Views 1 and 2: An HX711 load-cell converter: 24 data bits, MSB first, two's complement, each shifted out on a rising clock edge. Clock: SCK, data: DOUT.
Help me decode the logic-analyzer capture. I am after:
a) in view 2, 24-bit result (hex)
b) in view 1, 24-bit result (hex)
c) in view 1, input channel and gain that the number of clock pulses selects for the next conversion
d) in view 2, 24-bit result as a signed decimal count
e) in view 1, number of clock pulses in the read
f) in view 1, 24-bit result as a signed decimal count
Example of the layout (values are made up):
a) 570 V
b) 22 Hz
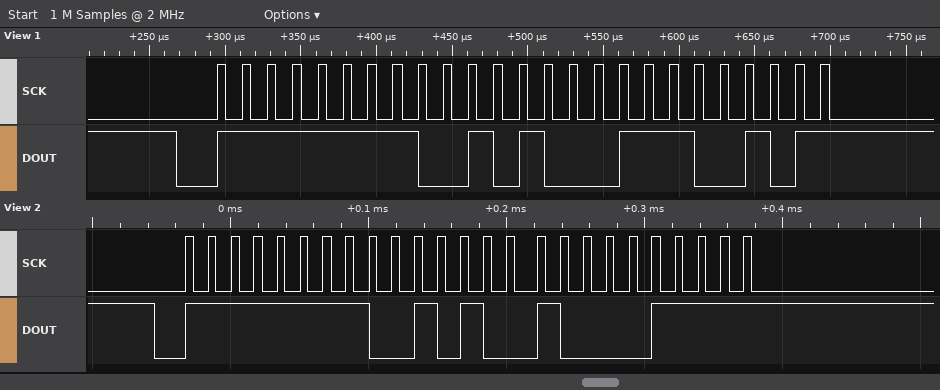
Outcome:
a) 0xFF290F
b) 0xFF28E5
c) channel A, gain 128
d) -55025
e) 25
f) -55067
